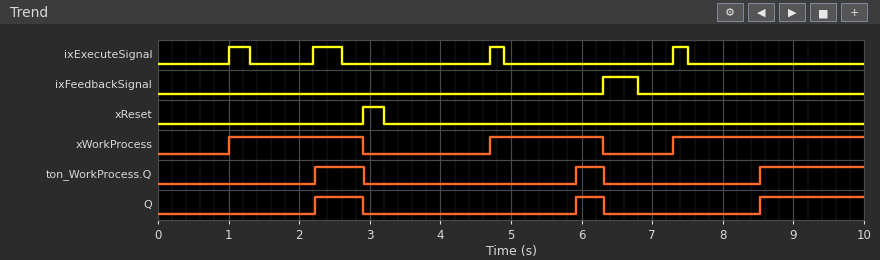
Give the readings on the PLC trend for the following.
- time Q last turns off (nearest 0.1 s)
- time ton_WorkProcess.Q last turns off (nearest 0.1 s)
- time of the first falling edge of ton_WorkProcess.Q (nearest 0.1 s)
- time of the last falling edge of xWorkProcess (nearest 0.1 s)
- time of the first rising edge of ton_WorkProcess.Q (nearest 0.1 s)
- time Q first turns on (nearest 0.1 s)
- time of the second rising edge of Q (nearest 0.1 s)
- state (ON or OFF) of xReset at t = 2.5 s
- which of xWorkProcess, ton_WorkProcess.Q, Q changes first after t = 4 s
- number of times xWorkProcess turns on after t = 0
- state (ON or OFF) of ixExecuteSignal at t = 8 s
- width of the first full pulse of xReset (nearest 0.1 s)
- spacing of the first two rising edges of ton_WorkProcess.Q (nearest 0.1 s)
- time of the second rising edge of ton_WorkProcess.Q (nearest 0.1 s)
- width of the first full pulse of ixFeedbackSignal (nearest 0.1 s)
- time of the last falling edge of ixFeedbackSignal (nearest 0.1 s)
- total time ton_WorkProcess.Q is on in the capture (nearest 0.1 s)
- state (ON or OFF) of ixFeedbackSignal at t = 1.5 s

6.3 s
6.3 s
2.9 s
6.3 s
2.2 s
2.2 s
5.9 s
OFF
xWorkProcess
3
OFF
0.3 s
3.7 s
5.9 s
0.5 s
6.8 s
2.6 s
OFF
